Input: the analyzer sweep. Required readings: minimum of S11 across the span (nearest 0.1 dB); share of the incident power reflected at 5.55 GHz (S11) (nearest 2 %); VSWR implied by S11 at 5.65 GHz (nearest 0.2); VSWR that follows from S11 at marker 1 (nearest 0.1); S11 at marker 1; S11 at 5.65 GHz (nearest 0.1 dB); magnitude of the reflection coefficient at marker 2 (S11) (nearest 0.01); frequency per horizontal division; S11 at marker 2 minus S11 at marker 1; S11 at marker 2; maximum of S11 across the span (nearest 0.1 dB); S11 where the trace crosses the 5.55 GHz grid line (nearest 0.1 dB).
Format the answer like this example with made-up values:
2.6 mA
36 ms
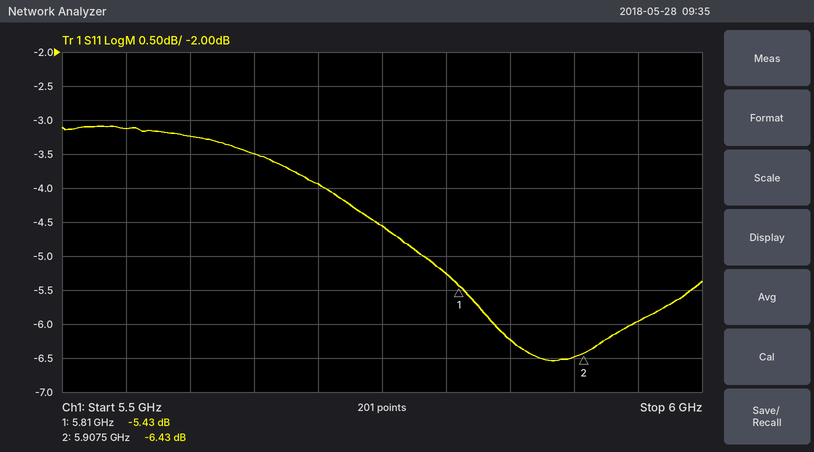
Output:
-6.5 dB
48 %
5.0
3.3
-5.43 dB
-3.5 dB
0.48
50 MHz
-1.00 dB
-6.43 dB
-3.1 dB
-3.1 dB
